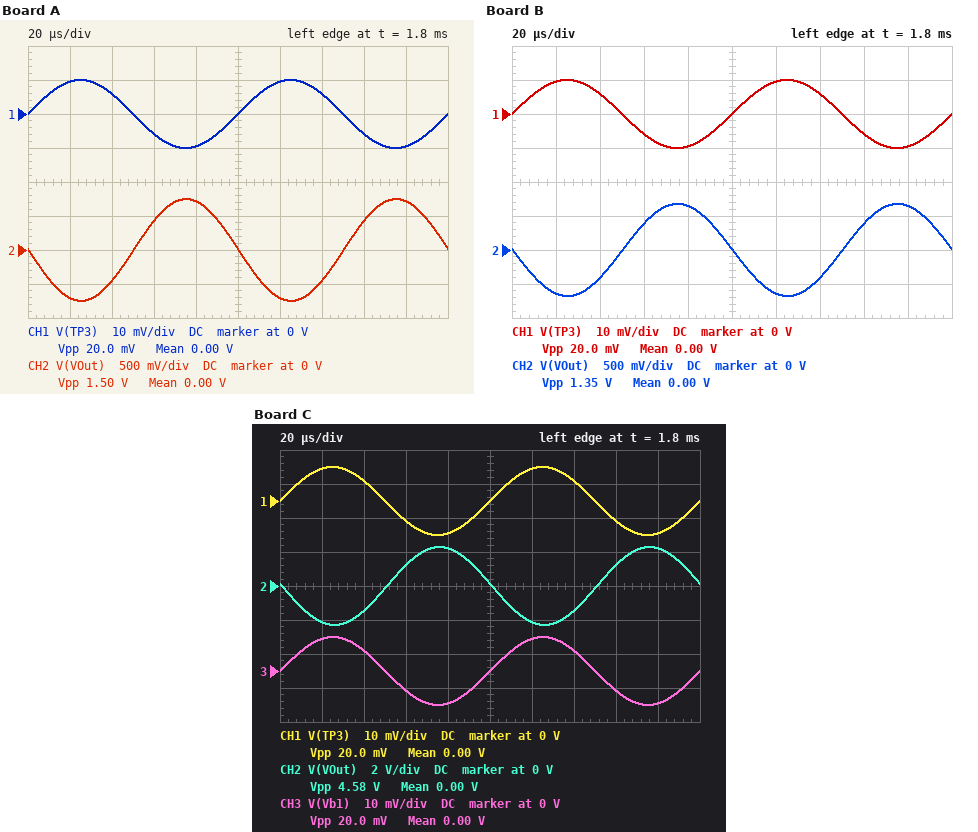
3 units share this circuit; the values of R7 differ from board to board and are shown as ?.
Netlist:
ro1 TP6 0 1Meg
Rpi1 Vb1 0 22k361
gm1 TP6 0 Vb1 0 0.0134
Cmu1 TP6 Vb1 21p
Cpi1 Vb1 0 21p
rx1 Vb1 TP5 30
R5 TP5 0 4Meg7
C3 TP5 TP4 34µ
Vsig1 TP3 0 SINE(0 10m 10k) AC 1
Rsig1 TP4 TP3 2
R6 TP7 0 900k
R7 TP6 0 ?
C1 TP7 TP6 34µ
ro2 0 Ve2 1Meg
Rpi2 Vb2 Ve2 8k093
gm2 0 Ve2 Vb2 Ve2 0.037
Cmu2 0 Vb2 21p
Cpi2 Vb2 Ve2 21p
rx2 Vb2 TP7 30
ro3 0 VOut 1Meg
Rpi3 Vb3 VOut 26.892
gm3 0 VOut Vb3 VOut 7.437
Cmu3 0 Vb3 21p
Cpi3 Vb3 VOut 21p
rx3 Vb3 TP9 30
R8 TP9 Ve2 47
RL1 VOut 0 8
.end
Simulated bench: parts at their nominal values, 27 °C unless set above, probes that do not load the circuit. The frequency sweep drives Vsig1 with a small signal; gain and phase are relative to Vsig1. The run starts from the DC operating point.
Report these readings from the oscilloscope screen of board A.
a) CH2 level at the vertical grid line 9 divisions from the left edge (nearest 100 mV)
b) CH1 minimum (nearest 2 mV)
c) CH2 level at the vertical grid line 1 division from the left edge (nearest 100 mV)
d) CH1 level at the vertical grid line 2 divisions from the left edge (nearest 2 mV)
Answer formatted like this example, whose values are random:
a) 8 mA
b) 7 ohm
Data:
a) 700 mV
b) -10 mV
c) -700 mV
d) 6 mV
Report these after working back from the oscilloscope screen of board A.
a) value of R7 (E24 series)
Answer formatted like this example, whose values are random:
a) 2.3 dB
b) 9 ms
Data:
a) 6.2 kΩ
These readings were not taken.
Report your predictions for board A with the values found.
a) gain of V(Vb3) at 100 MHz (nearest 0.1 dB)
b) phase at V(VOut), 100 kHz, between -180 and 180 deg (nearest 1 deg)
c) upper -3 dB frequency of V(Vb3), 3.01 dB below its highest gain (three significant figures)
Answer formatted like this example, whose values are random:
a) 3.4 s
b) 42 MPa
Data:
a) -12.0 dB
b) 169 deg
c) 511 kHz
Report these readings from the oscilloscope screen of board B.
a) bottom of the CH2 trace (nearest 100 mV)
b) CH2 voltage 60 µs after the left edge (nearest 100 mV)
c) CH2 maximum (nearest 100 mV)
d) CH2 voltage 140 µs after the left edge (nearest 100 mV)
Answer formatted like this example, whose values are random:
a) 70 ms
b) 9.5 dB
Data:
a) -700 mV
b) 400 mV
c) 700 mV
d) -400 mV
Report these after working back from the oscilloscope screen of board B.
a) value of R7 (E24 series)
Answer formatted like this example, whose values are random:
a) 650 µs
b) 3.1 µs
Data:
a) 5.6 kΩ
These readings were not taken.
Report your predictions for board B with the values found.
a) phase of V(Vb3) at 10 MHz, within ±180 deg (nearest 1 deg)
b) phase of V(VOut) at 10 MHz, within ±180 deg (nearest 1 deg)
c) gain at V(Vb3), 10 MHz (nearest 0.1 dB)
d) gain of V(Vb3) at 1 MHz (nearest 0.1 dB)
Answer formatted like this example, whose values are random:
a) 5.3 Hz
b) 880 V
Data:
a) 75 deg
b) 75 deg
c) 11.7 dB
d) 30.6 dB
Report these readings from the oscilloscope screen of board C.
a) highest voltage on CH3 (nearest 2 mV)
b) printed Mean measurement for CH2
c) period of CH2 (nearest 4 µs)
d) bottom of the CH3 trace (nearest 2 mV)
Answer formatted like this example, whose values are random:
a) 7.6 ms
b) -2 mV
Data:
a) 10 mV
b) 0.00 V
c) 100 µs
d) -10 mV
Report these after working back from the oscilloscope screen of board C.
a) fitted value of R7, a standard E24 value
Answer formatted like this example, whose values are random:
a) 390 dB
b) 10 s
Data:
a) 20 kΩ
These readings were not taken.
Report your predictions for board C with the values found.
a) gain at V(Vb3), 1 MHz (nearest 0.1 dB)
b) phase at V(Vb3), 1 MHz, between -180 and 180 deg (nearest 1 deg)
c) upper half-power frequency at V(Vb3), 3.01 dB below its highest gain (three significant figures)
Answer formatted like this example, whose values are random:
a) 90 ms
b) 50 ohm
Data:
a) 31.7 dB
b) 98 deg
c) 167 kHz
